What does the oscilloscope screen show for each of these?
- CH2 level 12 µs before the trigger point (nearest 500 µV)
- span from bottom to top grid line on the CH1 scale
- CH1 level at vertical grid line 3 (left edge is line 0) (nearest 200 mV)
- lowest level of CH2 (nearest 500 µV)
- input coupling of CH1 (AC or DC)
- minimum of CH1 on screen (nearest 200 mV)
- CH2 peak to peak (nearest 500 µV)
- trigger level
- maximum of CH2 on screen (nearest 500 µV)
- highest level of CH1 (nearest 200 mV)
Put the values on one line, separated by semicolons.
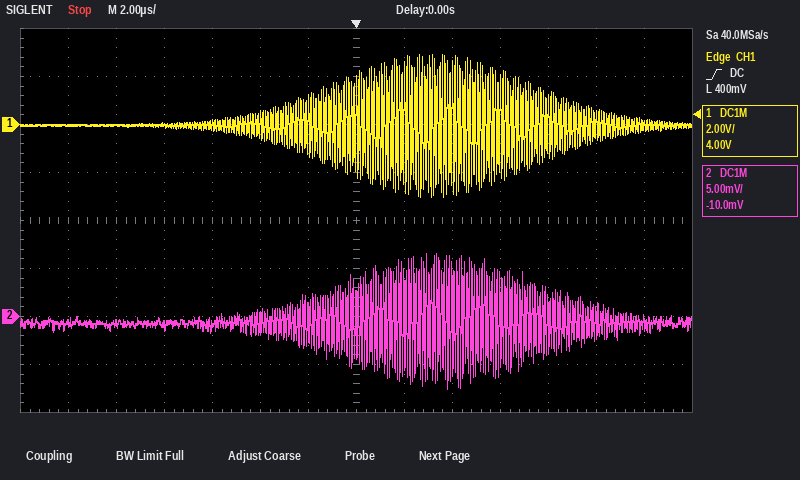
-500 µV; 16 V; 0.0 V; -7.5 mV; DC; -3.0 V; 14.0 mV; 400 mV; 6.5 mV; 3.0 V
